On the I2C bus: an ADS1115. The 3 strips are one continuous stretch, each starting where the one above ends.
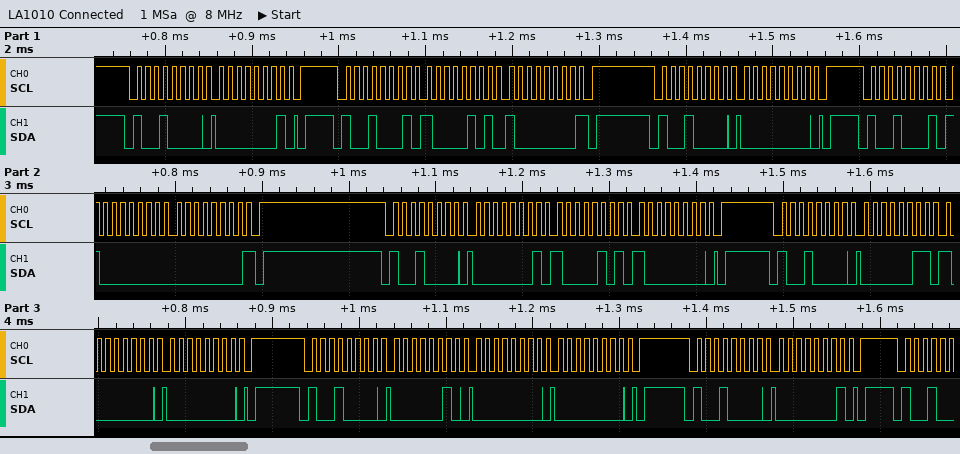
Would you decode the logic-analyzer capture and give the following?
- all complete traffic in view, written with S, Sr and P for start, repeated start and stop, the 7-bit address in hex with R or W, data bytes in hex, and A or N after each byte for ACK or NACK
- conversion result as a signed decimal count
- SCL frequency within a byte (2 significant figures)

S 48W A 01 A P S 48R A 85 A 80 N P S 48W A 00 A P S 48R A 80 A 00 N P S 48W A 01 A 85 A 80 A P S 48W A 03 A 80 A 00 A P S 48W A 02 A 00 A 00 A P S 48W A 01 A P
-32768
100 kHz
